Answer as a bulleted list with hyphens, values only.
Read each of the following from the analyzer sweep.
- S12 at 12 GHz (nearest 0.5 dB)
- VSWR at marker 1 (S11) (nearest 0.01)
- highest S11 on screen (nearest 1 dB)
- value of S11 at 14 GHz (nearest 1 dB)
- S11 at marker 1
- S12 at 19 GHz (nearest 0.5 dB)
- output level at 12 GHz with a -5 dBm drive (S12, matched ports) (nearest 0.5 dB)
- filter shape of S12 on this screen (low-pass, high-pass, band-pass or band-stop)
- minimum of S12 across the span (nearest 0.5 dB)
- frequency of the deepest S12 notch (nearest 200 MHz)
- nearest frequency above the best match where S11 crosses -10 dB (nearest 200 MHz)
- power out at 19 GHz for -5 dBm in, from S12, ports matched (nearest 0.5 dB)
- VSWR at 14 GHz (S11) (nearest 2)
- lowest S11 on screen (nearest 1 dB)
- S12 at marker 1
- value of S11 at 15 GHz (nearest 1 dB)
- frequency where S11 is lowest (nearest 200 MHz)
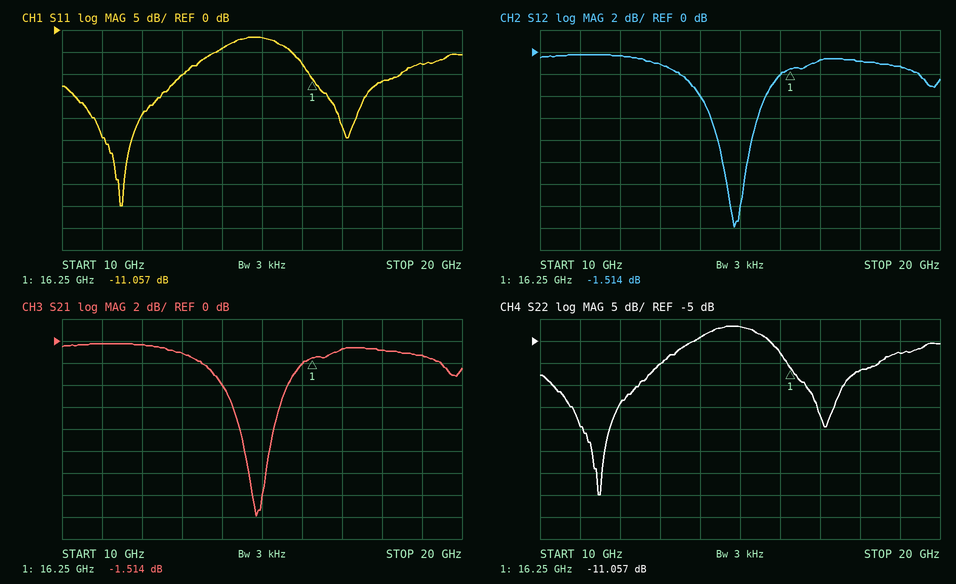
- -0.5 dB
- 1.78
- -2 dB
- -4 dB
- -11.057 dB
- -1.5 dB
- -5.5 dBm
- band-stop
- -16.0 dB
- 14.8 GHz
- 13.0 GHz
- -6.5 dBm
- 4
- -40 dB
- -1.514 dB
- -2 dB
- 11.4 GHz
